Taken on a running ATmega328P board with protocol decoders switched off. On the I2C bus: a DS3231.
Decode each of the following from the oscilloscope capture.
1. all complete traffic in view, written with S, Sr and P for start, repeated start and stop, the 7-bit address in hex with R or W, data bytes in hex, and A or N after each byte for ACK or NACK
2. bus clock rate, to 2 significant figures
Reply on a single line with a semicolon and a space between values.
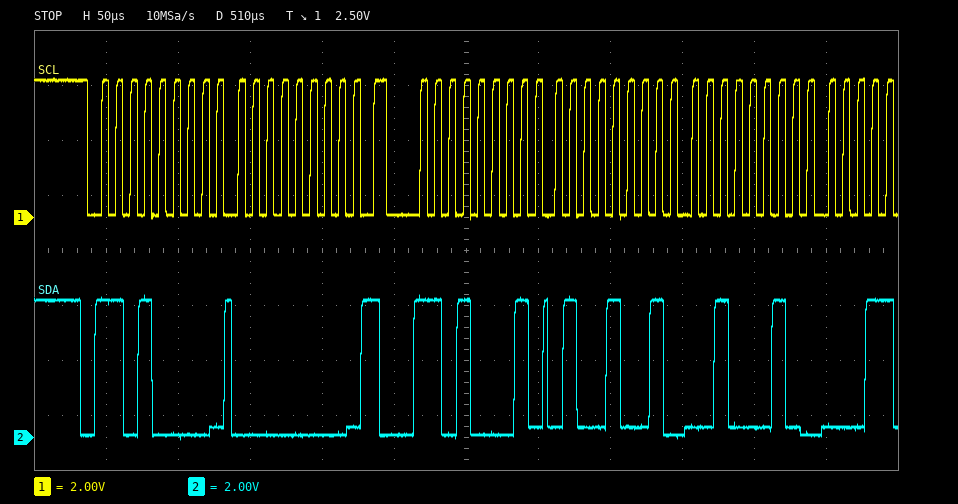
S 68W A 00 A Sr 68R A 49 A 22 A; 100 kHz
